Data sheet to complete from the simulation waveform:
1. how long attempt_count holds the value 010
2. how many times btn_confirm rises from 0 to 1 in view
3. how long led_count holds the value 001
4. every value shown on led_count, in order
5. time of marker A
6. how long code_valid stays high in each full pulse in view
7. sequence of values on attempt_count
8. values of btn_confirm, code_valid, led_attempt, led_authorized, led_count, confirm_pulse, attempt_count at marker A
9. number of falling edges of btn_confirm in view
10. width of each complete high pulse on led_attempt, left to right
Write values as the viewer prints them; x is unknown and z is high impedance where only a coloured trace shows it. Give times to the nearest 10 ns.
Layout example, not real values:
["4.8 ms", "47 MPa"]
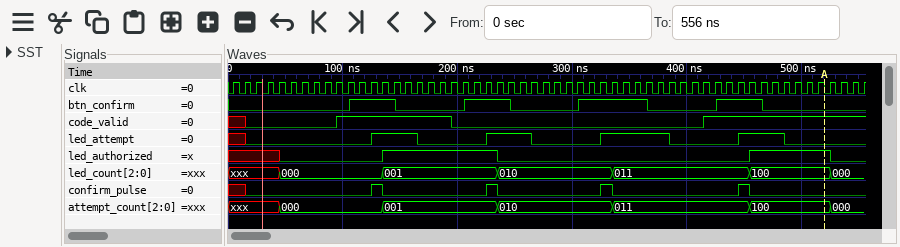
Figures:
["100 ns", "4", "100 ns", "xxx, 000, 001, 010, 011, 100, 000", "520 ns", "100 ns", "xxx, 000, 001, 010, 011, 100, 000", "btn_confirm=0, code_valid=1, led_attempt=0, led_authorized=1, led_count=100, confirm_pulse=0, attempt_count=100", "4", "40 ns, 40 ns, 60 ns, 40 ns"]
